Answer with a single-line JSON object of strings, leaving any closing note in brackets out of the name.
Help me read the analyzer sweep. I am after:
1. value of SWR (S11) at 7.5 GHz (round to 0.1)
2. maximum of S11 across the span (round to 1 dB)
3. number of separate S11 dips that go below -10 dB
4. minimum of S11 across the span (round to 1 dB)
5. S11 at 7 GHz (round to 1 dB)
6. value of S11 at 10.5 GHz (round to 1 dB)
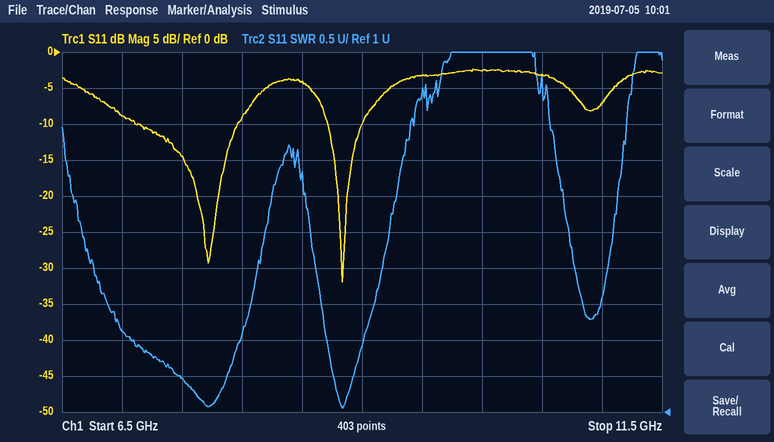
{"value of SWR (S11) at 7.5 GHz": "1.5", "maximum of S11 across the span": "-2 dB", "number of separate S11 dips that go below -10 dB": "2", "minimum of S11 across the span": "-32 dB", "S11 at 7 GHz": "-9 dB", "value of S11 at 10.5 GHz": "-3 dB"}
